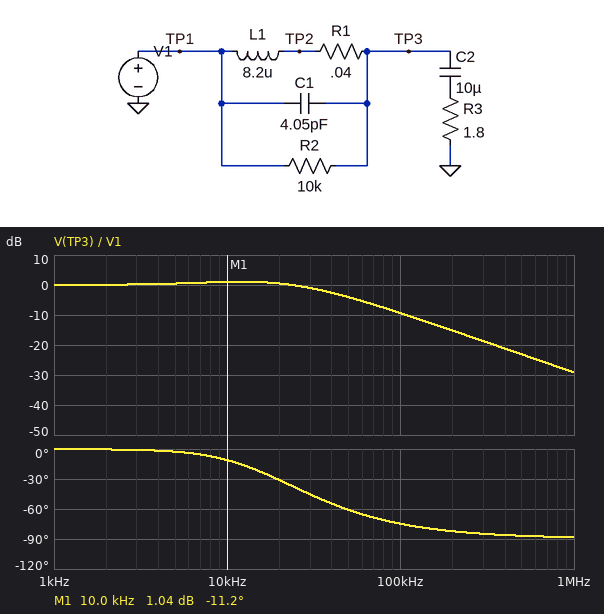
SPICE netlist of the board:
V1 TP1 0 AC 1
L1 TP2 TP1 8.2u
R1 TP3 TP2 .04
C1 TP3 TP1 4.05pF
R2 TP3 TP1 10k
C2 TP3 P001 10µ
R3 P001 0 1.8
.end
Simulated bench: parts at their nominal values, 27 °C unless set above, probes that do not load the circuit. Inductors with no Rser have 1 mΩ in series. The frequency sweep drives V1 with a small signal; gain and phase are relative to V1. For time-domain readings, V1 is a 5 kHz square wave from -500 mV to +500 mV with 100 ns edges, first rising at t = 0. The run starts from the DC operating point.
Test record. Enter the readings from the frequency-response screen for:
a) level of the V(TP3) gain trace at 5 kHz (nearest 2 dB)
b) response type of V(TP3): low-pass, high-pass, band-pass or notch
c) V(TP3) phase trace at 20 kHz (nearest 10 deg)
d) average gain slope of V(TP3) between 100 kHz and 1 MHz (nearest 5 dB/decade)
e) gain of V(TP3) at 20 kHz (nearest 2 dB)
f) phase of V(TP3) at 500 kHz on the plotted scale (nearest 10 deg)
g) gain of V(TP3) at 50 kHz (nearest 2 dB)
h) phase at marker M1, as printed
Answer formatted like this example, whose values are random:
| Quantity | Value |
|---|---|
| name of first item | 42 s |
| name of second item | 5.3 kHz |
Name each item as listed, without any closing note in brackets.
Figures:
| Quantity | Value |
|---|---|
| level of the V(TP3) gain trace at 5 kHz | 0 dB |
| response type of V(TP3): low-pass, high-pass, band-pass or notch | low-pass |
| V(TP3) phase trace at 20 kHz | -30 deg |
| average gain slope of V(TP3) between 100 kHz and 1 MHz | -20 dB/decade |
| gain of V(TP3) at 20 kHz | 0 dB |
| phase of V(TP3) at 500 kHz on the plotted scale | -90 deg |
| gain of V(TP3) at 50 kHz | -4 dB |
| phase at marker M1, as printed | -11.2 deg |
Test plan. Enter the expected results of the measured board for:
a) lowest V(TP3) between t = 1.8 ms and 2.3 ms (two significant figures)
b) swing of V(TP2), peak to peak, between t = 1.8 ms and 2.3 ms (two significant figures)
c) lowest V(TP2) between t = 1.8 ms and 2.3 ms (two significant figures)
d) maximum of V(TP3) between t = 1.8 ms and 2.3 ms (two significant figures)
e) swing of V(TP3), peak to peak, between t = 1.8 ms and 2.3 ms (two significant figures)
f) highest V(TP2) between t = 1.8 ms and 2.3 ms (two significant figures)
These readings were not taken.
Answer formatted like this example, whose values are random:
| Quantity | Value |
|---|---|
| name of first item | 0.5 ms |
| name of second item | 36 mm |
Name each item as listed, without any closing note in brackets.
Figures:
| Quantity | Value |
|---|---|
| lowest V(TP3) between t = 1.8 ms and 2.3 ms | -620 mV |
| swing of V(TP2), peak to peak, between t = 1.8 ms and 2.3 ms | 1.3 V |
| lowest V(TP2) between t = 1.8 ms and 2.3 ms | -630 mV |
| maximum of V(TP3) between t = 1.8 ms and 2.3 ms | 620 mV |
| swing of V(TP3), peak to peak, between t = 1.8 ms and 2.3 ms | 1.2 V |
| highest V(TP2) between t = 1.8 ms and 2.3 ms | 630 mV |
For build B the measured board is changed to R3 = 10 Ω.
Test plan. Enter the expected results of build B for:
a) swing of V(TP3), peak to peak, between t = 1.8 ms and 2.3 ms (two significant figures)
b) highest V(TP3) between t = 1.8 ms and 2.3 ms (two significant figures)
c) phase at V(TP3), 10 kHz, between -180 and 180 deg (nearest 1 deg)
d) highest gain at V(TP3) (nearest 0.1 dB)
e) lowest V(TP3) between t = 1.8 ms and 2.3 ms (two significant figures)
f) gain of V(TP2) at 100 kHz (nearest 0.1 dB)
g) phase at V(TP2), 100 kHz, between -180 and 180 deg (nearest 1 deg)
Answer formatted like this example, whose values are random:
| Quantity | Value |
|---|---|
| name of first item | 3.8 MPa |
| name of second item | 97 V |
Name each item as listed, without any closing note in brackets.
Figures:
| Quantity | Value |
|---|---|
| swing of V(TP3), peak to peak, between t = 1.8 ms and 2.3 ms | 1.0 V |
| highest V(TP3) between t = 1.8 ms and 2.3 ms | 500 mV |
| phase at V(TP3), 10 kHz, between -180 and 180 deg | -3 deg |
| highest gain at V(TP3) | 0 dB |
| lowest V(TP3) between t = 1.8 ms and 2.3 ms | -500 mV |
| gain of V(TP2) at 100 kHz | -1.0 dB |
| phase at V(TP2), 100 kHz, between -180 and 180 deg | -27 deg |
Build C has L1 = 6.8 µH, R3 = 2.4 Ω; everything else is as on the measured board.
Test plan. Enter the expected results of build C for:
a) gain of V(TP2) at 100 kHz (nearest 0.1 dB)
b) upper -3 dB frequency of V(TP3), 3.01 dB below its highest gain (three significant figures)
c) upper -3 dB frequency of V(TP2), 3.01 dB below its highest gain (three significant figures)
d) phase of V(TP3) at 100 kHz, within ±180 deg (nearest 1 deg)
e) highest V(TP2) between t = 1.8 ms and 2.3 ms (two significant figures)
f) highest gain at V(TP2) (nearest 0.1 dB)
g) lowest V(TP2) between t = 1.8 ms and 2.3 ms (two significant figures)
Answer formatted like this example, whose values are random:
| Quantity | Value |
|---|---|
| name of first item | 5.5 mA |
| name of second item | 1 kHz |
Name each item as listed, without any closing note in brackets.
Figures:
| Quantity | Value |
|---|---|
| gain of V(TP2) at 100 kHz | -5.8 dB |
| upper -3 dB frequency of V(TP3), 3.01 dB below its highest gain | 55.4 kHz |
| upper -3 dB frequency of V(TP2), 3.01 dB below its highest gain | 55.8 kHz |
| phase of V(TP3) at 100 kHz, within ±180 deg | -63 deg |
| highest V(TP2) between t = 1.8 ms and 2.3 ms | 580 mV |
| highest gain at V(TP2) | 0.7 dB |
| lowest V(TP2) between t = 1.8 ms and 2.3 ms | -580 mV |
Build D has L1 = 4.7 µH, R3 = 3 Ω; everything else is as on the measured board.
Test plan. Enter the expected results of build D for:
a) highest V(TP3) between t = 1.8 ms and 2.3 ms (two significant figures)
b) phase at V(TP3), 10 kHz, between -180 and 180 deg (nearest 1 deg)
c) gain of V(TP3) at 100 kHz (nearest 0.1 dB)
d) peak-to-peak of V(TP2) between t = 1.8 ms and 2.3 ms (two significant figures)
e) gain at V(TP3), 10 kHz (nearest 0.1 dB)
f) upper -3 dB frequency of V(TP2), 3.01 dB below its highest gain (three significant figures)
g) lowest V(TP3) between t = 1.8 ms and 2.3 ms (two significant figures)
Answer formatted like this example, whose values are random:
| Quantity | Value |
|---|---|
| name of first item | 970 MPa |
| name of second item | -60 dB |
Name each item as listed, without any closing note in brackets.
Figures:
| Quantity | Value |
|---|---|
| highest V(TP3) between t = 1.8 ms and 2.3 ms | 530 mV |
| phase at V(TP3), 10 kHz, between -180 and 180 deg | -5 deg |
| gain of V(TP3) at 100 kHz | -2.8 dB |
| peak-to-peak of V(TP2) between t = 1.8 ms and 2.3 ms | 1.1 V |
| gain at V(TP3), 10 kHz | 0.2 dB |
| upper -3 dB frequency of V(TP2), 3.01 dB below its highest gain | 101 kHz |
| lowest V(TP3) between t = 1.8 ms and 2.3 ms | -530 mV |
